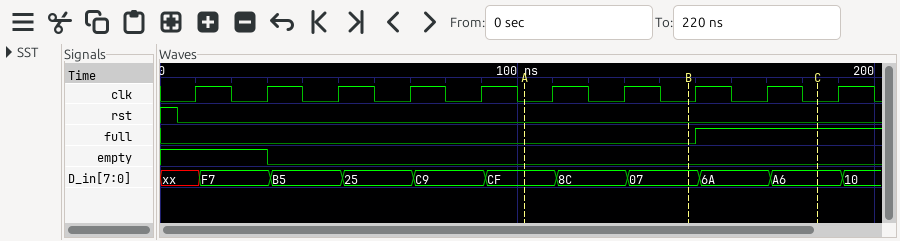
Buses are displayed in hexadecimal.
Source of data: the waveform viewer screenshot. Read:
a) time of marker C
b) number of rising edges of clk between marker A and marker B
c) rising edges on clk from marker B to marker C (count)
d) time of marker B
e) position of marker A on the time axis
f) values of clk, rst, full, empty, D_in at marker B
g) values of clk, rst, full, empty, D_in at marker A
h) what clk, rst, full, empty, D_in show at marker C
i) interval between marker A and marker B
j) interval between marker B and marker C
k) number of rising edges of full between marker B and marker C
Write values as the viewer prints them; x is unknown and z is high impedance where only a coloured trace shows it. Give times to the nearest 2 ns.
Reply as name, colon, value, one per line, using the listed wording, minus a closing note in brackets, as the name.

time of marker C: 184 ns
number of rising edges of clk between marker A and marker B: 2
rising edges on clk from marker B to marker C: 2
time of marker B: 148 ns
position of marker A on the time axis: 102 ns
values of clk, rst, full, empty, D_in at marker B: clk=0, rst=0, full=0, empty=0, D_in=07
values of clk, rst, full, empty, D_in at marker A: clk=0, rst=0, full=0, empty=0, D_in=CF
what clk, rst, full, empty, D_in show at marker C: clk=0, rst=0, full=1, empty=0, D_in=A6
interval between marker A and marker B: 46 ns
interval between marker B and marker C: 36 ns
number of rising edges of full between marker B and marker C: 1
